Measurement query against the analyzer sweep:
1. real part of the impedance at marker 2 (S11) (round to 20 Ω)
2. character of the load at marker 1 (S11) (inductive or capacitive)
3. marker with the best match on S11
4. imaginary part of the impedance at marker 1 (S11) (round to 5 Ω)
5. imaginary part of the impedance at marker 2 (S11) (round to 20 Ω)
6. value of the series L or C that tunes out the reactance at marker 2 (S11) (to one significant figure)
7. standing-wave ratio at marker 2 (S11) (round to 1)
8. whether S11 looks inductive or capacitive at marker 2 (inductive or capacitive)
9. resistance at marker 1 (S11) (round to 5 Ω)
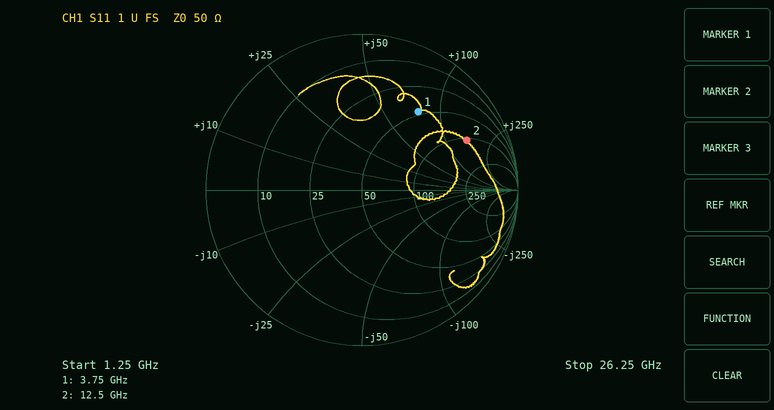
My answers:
100 Ω
inductive
marker 1
+75 Ω
+160 Ω
80 fF
7
inductive
45 Ω
